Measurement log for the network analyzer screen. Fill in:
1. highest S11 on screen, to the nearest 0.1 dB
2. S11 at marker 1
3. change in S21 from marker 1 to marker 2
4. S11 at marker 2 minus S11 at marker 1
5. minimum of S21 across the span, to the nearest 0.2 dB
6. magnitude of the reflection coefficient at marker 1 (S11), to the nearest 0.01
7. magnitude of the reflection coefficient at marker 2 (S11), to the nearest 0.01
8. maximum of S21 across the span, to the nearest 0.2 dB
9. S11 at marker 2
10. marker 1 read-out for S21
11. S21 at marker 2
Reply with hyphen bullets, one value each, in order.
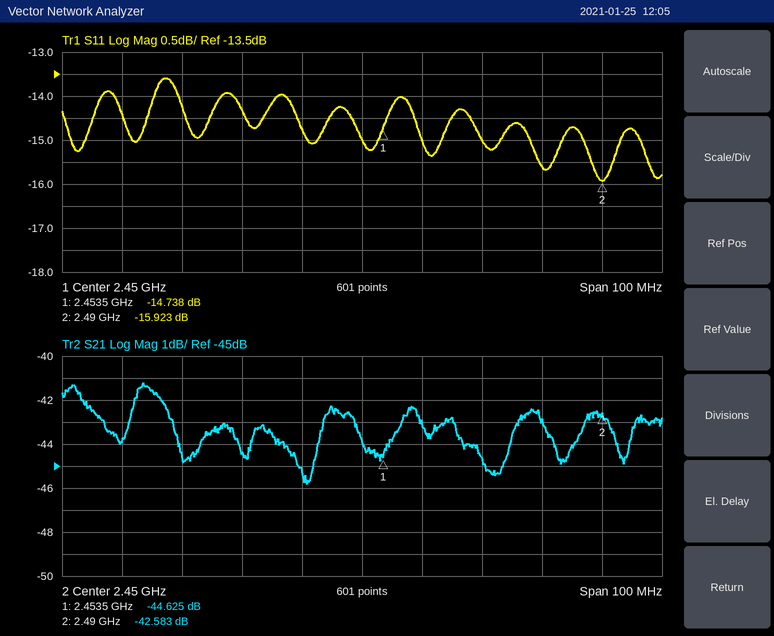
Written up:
- -13.6 dB
- -14.738 dB
- 2.042 dB
- -1.185 dB
- -45.8 dB
- 0.18
- 0.16
- -41.2 dB
- -15.923 dB
- -44.625 dB
- -42.583 dB
